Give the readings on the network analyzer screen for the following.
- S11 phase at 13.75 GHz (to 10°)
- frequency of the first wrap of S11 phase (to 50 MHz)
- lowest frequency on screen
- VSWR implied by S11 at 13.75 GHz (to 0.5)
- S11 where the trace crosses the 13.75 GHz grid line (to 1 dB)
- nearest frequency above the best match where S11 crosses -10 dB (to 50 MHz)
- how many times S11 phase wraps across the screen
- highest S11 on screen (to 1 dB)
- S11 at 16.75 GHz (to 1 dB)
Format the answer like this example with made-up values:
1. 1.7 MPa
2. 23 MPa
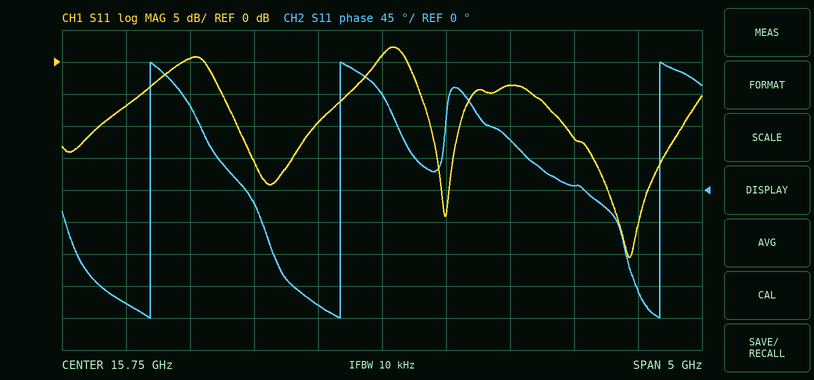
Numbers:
1. -160°
2. 13.95 GHz
3. 13.25 GHz
4. 2.5
5. -7 dB
6. 18.10 GHz
7. 3
8. 2 dB
9. -4 dB
